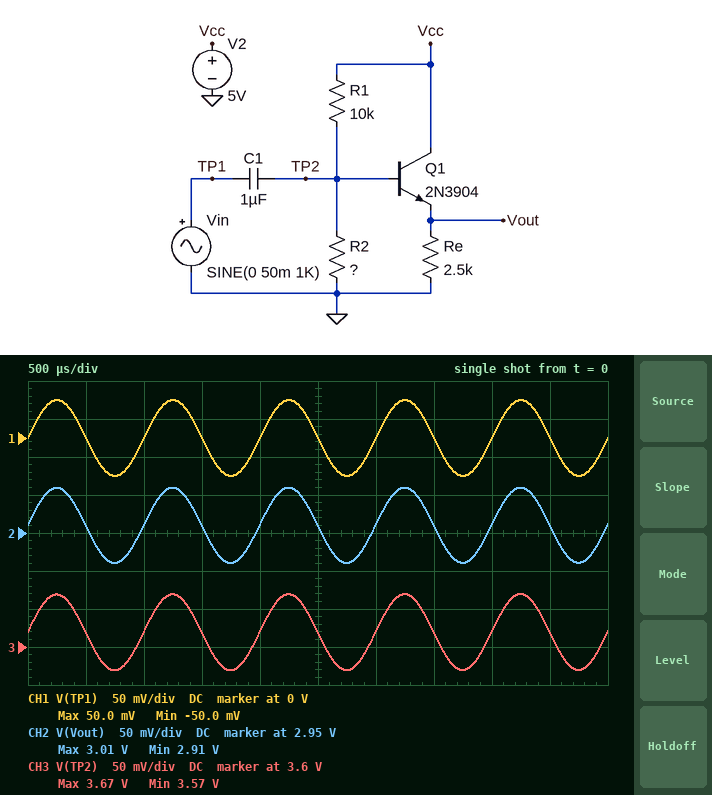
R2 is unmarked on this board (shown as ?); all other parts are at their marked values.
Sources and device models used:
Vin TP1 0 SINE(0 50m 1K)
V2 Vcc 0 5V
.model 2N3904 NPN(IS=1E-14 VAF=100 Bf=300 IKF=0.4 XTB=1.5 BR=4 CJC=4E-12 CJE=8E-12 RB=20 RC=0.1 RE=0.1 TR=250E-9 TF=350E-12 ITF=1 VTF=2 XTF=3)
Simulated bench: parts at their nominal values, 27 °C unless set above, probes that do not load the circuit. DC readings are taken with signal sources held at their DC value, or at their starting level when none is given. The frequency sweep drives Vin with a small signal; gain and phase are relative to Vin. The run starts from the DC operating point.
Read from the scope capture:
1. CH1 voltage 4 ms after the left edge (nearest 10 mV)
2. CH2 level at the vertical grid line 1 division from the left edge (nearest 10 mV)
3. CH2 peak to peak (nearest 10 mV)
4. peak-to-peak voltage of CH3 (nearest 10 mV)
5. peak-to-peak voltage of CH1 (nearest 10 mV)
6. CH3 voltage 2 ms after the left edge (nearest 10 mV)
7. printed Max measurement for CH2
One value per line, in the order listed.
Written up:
0 V
2.96 V
100 mV
100 mV
100 mV
3.62 V
3.01 V
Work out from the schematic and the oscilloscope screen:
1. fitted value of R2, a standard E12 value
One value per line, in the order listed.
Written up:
27 kΩ
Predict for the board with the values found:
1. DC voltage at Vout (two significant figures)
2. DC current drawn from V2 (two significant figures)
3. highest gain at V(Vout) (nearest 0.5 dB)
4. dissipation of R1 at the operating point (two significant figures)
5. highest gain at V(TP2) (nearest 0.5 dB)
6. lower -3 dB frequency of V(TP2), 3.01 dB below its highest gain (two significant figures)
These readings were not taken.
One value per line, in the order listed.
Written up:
3.0 V
1.3 mA
0 dB
190 µW
0 dB
22 Hz
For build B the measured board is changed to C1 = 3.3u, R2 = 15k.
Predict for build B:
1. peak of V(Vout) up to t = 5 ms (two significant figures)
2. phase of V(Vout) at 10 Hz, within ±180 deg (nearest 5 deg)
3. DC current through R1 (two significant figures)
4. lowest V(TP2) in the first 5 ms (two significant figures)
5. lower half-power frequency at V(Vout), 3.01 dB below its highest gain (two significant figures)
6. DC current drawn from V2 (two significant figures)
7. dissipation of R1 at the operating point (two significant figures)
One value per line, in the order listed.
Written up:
2.4 V
40 deg
200 µA
2.9 V
8.1 Hz
1.1 mA
410 µW
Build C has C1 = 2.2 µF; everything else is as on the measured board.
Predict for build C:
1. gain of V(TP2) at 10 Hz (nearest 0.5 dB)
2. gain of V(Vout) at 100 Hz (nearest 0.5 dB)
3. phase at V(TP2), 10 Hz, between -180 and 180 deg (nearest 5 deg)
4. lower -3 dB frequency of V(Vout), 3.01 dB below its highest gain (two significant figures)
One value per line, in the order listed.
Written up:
-3.0 dB
0 dB
45 deg
10 Hz
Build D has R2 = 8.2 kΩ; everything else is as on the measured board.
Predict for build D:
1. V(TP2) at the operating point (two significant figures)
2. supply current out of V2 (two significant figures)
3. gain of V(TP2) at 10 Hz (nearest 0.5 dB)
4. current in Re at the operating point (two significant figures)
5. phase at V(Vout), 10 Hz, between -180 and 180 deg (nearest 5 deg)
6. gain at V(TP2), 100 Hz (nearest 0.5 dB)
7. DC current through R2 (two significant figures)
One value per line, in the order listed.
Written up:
2.2 V
910 µA
-11.5 dB
640 µA
75 deg
-0.5 dB
270 µA
